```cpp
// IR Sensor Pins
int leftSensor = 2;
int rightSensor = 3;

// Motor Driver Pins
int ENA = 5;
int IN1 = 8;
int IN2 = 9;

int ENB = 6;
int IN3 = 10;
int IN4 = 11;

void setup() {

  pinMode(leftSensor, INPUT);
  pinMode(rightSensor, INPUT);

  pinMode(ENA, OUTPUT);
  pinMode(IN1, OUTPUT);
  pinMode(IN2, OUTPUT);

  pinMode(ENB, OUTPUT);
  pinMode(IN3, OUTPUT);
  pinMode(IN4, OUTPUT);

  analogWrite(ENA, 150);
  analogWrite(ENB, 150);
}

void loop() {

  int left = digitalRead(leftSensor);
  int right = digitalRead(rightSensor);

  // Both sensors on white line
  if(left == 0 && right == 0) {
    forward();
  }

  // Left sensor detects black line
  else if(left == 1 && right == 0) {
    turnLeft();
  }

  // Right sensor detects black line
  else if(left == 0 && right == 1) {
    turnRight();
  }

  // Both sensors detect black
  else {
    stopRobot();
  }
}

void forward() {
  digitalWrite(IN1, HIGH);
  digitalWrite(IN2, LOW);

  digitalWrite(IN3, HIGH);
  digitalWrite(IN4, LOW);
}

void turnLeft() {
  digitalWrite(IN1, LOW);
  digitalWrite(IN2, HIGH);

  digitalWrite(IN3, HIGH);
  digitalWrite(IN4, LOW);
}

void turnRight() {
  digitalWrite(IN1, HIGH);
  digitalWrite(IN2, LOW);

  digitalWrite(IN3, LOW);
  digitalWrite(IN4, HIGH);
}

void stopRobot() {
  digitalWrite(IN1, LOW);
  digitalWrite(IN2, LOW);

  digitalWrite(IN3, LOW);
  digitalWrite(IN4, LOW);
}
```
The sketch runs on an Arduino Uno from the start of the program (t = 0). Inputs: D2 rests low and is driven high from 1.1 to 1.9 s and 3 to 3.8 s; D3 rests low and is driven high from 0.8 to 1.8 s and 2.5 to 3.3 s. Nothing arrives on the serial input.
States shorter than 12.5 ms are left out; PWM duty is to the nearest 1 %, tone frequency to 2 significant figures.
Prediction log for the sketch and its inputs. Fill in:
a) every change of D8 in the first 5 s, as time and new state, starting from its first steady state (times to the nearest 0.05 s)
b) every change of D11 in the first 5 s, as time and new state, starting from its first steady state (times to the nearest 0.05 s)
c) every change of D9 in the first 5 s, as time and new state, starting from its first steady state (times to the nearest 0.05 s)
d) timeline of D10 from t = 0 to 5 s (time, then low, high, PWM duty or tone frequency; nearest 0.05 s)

0 s high; 1.1 s low; 1.9 s high; 3 s low; 3.8 s high
0 s low; 0.8 s high; 1.1 s low; 2.5 s high; 3 s low
0 s low; 1.8 s high; 1.9 s low; 3.3 s high; 3.8 s low
0 s high; 0.8 s low; 1.8 s high; 2.5 s low; 3.3 s high
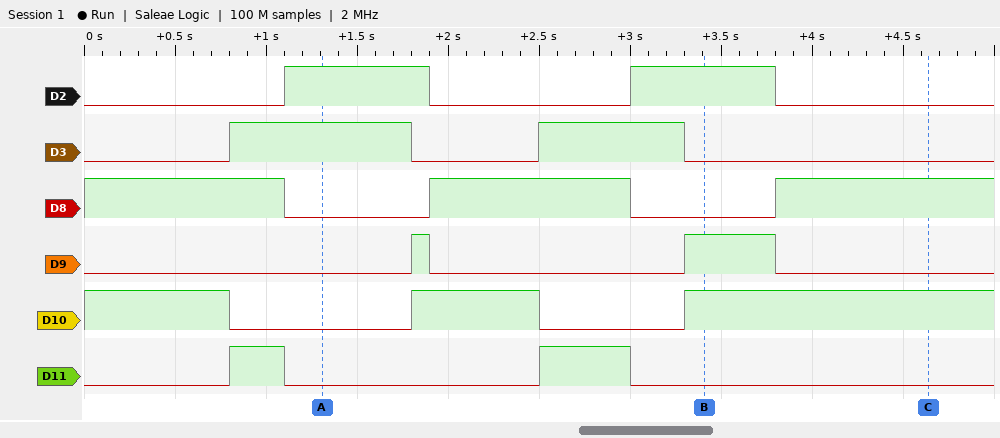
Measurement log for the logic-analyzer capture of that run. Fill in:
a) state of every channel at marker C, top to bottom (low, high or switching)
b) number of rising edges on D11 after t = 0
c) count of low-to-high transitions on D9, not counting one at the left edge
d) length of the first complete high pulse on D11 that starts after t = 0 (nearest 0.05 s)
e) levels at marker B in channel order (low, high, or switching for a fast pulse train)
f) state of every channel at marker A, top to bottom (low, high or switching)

D2 low, D3 low, D8 high, D9 low, D10 high, D11 low
2
2
0.30 s
D2 high, D3 low, D8 low, D9 high, D10 high, D11 low
D2 high, D3 high, D8 low, D9 low, D10 low, D11 low
